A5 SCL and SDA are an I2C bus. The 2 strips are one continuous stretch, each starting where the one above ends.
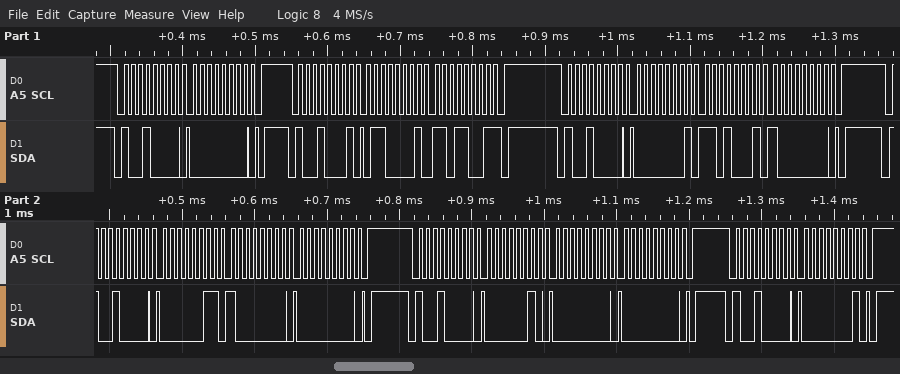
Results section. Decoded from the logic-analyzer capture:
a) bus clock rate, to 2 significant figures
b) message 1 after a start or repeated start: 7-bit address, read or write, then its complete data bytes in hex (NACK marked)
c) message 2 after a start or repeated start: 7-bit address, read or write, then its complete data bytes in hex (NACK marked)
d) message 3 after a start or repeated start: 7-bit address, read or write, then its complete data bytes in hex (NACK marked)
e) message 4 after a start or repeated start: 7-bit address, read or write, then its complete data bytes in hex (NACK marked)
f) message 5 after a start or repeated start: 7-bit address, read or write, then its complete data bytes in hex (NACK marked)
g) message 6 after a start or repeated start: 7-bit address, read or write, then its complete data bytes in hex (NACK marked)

100 kHz
0x48 write: 00
0x48 read: 61 D9 NACK
0x48 write: 01 D1 80
0x48 write: 03 80 00
0x48 write: 02 00 00
0x48 write: 01
